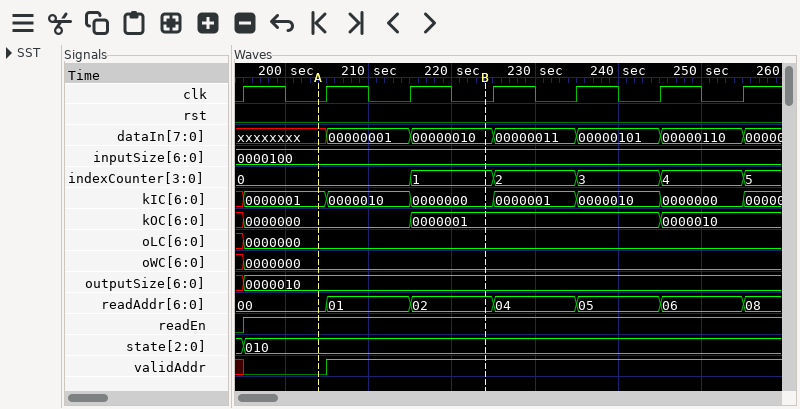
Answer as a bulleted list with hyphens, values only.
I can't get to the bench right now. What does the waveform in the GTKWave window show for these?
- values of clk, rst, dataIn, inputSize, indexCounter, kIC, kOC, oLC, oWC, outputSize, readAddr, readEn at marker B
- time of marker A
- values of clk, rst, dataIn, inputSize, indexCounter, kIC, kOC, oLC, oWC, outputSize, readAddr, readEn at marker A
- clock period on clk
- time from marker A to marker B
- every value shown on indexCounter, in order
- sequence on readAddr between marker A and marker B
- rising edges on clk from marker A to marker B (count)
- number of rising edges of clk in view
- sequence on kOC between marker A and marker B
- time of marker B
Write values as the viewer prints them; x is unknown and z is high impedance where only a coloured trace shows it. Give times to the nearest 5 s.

- clk=0, rst=0, dataIn=00000010, inputSize=0000100, indexCounter=1, kIC=0000000, kOC=0000001, oLC=0000000, oWC=0000000, outputSize=0000010, readAddr=02, readEn=1
- 205 s
- clk=0, rst=0, dataIn=xxxxxxxx, inputSize=0000100, indexCounter=0, kIC=0000001, kOC=0000000, oLC=0000000, oWC=0000000, outputSize=0000010, readAddr=00, readEn=1
- 10 s
- 20 s
- 0, 1, 2, 3, 4, 5
- 00, 01, 02
- 2
- 7
- 0000000, 0000001
- 225 s
